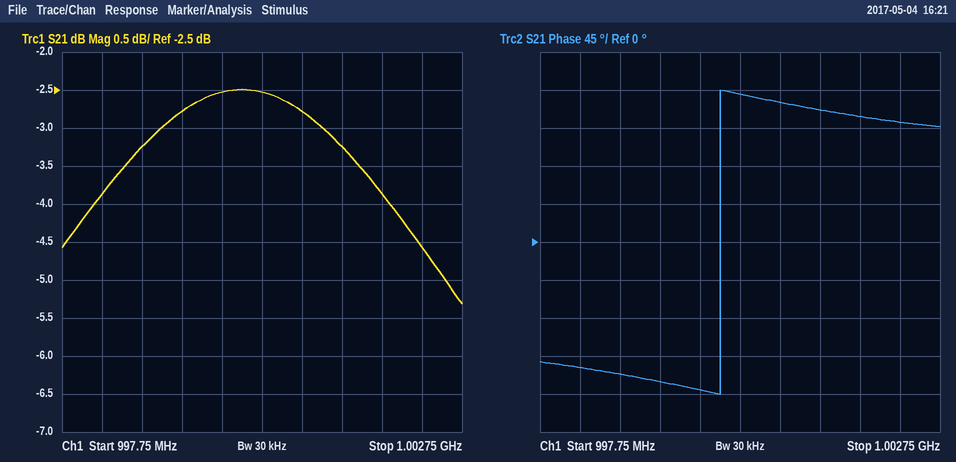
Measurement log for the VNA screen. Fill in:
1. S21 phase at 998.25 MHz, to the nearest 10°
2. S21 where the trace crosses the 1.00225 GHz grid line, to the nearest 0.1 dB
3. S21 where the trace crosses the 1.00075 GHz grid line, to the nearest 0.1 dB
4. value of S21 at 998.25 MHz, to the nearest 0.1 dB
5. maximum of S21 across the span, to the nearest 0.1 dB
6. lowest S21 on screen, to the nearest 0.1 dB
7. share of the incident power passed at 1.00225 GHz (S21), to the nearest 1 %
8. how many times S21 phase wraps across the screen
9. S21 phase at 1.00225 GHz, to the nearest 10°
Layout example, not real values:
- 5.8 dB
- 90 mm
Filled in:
- -150°
- -4.6 dB
- -2.8 dB
- -3.9 dB
- -2.5 dB
- -5.3 dB
- 35 %
- 1
- 140°
